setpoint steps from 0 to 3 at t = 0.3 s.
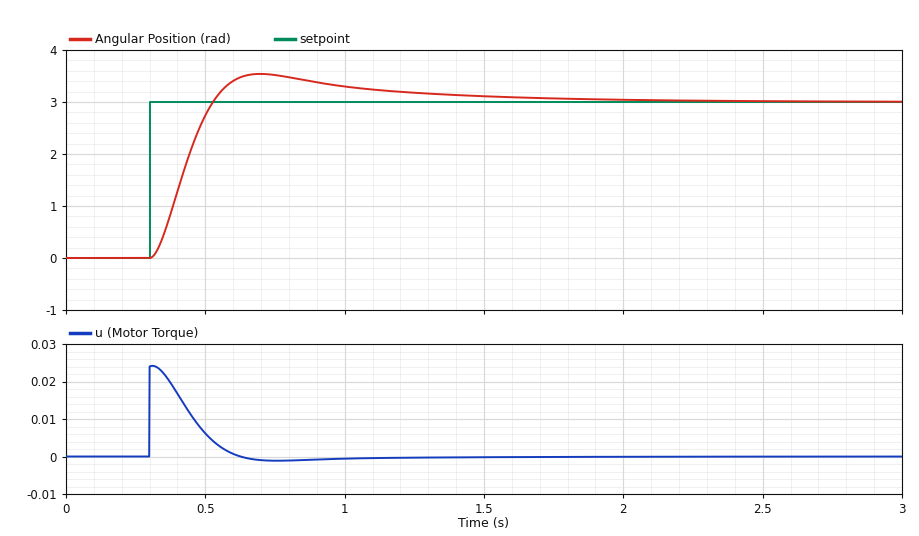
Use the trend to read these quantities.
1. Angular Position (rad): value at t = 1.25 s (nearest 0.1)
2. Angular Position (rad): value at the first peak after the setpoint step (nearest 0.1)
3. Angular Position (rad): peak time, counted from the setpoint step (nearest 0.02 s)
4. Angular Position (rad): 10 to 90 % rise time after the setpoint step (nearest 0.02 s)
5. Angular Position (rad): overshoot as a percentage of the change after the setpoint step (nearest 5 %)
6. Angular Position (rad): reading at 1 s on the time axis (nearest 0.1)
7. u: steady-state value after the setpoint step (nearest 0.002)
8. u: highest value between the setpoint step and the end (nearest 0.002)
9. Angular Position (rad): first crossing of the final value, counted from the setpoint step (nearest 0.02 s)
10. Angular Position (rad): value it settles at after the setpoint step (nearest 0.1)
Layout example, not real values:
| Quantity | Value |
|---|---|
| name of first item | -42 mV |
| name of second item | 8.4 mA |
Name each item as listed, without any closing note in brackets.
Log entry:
| Quantity | Value |
|---|---|
| Angular Position (rad): value at t = 1.25 s | 3.2 |
| Angular Position (rad): value at the first peak after the setpoint step | 3.5 |
| Angular Position (rad): peak time, counted from the setpoint step | 0.40 s |
| Angular Position (rad): 10 to 90 % rise time after the setpoint step | 0.16 s |
| Angular Position (rad): overshoot as a percentage of the change after the setpoint step | 20 % |
| Angular Position (rad): reading at 1 s on the time axis | 3.3 |
| u: steady-state value after the setpoint step | 0.000 |
| u: highest value between the setpoint step and the end | 0.024 |
| Angular Position (rad): first crossing of the final value, counted from the setpoint step | 0.22 s |
| Angular Position (rad): value it settles at after the setpoint step | 3.0 |
